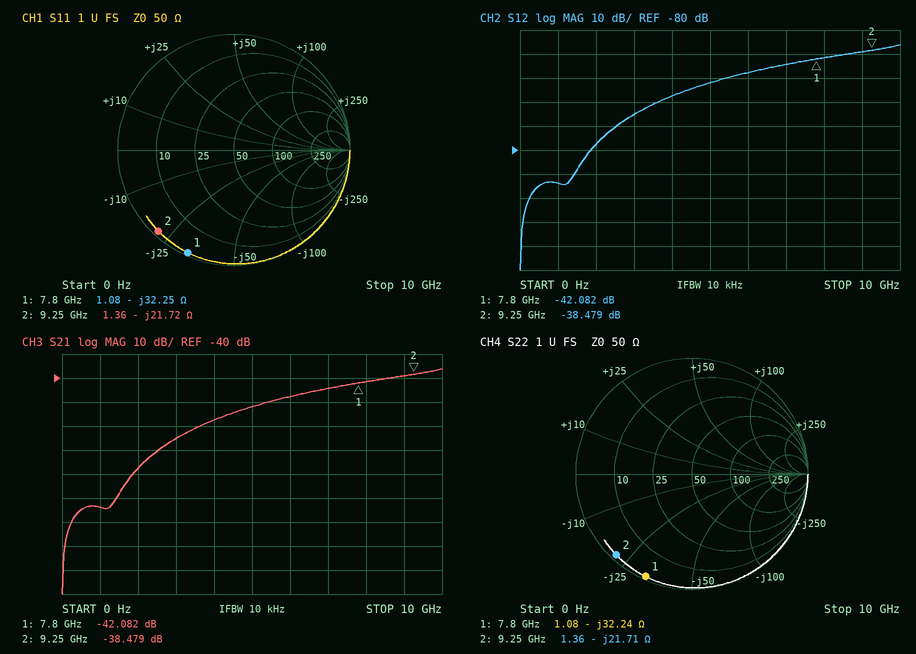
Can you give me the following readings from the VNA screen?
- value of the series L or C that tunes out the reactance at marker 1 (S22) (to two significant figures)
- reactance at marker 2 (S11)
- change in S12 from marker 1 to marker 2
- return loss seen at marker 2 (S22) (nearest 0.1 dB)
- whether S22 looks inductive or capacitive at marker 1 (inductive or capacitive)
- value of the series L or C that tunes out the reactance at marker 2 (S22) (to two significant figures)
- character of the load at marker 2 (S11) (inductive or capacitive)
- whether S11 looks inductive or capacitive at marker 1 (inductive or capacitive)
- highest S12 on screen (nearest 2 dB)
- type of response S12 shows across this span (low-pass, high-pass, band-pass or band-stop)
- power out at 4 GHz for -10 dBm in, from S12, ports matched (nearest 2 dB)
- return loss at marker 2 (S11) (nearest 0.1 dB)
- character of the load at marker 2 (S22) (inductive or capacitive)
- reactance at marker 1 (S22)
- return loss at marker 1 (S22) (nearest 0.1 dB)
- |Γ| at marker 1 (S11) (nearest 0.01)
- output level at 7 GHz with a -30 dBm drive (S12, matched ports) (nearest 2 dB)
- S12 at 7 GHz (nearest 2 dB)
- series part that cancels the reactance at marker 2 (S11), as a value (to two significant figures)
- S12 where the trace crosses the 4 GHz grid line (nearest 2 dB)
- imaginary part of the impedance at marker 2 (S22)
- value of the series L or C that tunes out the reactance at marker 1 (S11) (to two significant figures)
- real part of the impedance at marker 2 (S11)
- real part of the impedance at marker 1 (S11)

660 pH
-21.72 Ω
3.603 dB
0.4 dB
capacitive
370 pH
capacitive
capacitive
-36 dB
high-pass
-68 dBm
0.4 dB
capacitive
-32.24 Ω
0.3 dB
0.97
-74 dBm
-44 dB
370 pH
-58 dB
-21.71 Ω
660 pH
1.36 Ω
1.08 Ω
